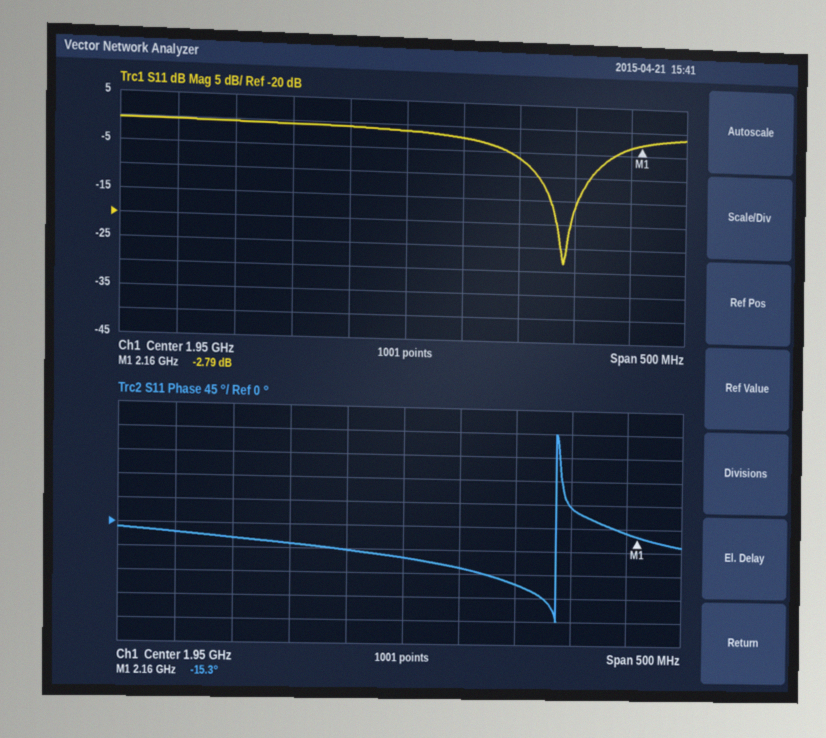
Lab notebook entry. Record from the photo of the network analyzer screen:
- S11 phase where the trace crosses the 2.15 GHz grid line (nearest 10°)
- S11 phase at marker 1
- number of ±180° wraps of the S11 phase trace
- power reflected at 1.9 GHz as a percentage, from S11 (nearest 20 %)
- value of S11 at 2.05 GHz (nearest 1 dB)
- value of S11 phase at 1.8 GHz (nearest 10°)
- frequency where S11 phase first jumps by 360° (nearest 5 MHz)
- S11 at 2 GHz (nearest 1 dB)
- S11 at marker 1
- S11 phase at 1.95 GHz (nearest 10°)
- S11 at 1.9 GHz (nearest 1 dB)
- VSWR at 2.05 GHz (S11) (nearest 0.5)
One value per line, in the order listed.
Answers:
-10°
-15.3°
1
80 %
-6 dB
-30°
2.085 GHz
-2 dB
-2.79 dB
-60°
-1 dB
3.0
